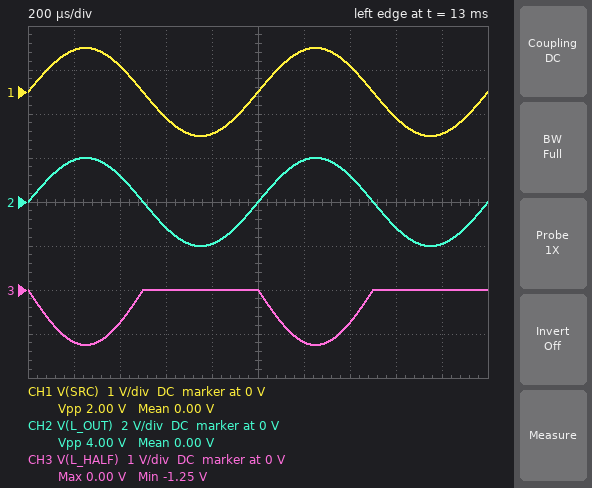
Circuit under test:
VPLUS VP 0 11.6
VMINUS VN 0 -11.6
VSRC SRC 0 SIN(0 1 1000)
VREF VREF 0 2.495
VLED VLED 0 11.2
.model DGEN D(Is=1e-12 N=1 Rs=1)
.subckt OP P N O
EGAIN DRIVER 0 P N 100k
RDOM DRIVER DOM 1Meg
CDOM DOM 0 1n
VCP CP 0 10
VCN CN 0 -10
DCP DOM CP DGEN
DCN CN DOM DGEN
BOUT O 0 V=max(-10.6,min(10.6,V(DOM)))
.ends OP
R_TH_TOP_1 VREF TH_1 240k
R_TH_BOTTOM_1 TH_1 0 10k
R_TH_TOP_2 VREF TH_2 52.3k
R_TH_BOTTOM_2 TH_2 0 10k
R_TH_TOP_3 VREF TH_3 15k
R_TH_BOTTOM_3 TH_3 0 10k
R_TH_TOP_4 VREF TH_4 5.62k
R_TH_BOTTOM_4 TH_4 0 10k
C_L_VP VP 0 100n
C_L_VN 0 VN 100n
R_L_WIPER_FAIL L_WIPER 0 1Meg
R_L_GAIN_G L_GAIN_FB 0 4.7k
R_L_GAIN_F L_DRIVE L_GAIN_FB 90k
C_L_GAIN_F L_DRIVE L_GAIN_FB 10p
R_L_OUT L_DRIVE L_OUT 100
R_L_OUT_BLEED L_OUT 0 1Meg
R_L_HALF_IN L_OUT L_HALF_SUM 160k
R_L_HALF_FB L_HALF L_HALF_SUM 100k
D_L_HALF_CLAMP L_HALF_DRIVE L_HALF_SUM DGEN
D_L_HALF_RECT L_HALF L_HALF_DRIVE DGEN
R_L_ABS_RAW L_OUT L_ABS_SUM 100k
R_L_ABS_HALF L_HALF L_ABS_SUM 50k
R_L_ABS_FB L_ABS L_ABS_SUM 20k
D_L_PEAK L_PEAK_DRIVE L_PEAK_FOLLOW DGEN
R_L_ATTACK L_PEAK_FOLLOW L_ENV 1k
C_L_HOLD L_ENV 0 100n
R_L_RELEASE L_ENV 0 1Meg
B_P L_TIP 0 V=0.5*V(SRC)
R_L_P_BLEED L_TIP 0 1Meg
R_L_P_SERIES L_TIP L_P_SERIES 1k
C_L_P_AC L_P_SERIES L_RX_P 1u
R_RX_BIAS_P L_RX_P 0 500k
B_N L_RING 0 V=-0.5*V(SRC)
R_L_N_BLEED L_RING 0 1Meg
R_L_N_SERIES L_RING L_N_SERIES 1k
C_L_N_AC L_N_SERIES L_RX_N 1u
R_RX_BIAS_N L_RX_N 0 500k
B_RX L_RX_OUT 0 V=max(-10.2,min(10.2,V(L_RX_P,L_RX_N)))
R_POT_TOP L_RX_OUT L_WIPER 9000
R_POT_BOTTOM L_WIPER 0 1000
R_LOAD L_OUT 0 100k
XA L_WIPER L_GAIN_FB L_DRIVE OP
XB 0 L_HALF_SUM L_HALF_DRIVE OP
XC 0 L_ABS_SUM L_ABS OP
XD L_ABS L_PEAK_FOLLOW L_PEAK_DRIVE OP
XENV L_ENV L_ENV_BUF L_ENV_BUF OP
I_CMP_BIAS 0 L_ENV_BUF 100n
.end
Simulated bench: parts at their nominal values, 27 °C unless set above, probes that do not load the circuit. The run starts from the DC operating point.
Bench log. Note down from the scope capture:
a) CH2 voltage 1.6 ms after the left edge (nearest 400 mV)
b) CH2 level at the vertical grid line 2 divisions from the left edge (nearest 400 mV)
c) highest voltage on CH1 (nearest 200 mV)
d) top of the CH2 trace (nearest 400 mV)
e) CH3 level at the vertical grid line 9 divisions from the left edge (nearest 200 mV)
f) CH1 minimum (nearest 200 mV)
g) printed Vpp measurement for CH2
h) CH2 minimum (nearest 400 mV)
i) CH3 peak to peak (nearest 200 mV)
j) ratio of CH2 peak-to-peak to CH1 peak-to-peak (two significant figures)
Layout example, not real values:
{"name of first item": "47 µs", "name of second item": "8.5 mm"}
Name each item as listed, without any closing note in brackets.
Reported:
{"CH2 voltage 1.6 ms after the left edge": "-1.2 V", "CH2 level at the vertical grid line 2 divisions from the left edge": "1.2 V", "highest voltage on CH1": "1.0 V", "top of the CH2 trace": "2.0 V", "CH3 level at the vertical grid line 9 divisions from the left edge": "0 V", "CH1 minimum": "-1.0 V", "printed Vpp measurement for CH2": "4.00 V", "CH2 minimum": "-2.0 V", "CH3 peak to peak": "1.2 V", "ratio of CH2 peak-to-peak to CH1 peak-to-peak": "2.0"}
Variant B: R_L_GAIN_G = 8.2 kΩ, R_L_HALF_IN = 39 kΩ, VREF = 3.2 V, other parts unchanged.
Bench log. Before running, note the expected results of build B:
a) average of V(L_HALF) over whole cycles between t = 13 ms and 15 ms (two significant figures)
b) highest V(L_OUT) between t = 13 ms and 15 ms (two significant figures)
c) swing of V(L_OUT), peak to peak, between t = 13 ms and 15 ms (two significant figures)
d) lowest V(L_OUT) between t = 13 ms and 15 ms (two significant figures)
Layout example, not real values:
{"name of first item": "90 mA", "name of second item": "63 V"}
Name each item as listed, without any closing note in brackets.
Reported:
{"average of V(L_HALF) over whole cycles between t = 13 ms and 15 ms": "-970 mV", "highest V(L_OUT) between t = 13 ms and 15 ms": "1.2 V", "swing of V(L_OUT), peak to peak, between t = 13 ms and 15 ms": "2.4 V", "lowest V(L_OUT) between t = 13 ms and 15 ms": "-1.2 V"}
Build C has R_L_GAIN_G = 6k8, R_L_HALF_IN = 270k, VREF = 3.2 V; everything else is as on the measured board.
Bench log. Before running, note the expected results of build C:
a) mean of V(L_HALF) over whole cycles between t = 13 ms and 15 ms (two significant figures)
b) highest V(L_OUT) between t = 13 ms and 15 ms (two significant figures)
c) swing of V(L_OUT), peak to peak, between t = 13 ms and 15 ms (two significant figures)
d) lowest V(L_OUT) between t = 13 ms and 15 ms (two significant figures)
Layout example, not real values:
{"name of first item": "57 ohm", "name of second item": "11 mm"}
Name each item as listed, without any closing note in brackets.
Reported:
{"mean of V(L_HALF) over whole cycles between t = 13 ms and 15 ms": "-170 mV", "highest V(L_OUT) between t = 13 ms and 15 ms": "1.4 V", "swing of V(L_OUT), peak to peak, between t = 13 ms and 15 ms": "2.8 V", "lowest V(L_OUT) between t = 13 ms and 15 ms": "-1.4 V"}
